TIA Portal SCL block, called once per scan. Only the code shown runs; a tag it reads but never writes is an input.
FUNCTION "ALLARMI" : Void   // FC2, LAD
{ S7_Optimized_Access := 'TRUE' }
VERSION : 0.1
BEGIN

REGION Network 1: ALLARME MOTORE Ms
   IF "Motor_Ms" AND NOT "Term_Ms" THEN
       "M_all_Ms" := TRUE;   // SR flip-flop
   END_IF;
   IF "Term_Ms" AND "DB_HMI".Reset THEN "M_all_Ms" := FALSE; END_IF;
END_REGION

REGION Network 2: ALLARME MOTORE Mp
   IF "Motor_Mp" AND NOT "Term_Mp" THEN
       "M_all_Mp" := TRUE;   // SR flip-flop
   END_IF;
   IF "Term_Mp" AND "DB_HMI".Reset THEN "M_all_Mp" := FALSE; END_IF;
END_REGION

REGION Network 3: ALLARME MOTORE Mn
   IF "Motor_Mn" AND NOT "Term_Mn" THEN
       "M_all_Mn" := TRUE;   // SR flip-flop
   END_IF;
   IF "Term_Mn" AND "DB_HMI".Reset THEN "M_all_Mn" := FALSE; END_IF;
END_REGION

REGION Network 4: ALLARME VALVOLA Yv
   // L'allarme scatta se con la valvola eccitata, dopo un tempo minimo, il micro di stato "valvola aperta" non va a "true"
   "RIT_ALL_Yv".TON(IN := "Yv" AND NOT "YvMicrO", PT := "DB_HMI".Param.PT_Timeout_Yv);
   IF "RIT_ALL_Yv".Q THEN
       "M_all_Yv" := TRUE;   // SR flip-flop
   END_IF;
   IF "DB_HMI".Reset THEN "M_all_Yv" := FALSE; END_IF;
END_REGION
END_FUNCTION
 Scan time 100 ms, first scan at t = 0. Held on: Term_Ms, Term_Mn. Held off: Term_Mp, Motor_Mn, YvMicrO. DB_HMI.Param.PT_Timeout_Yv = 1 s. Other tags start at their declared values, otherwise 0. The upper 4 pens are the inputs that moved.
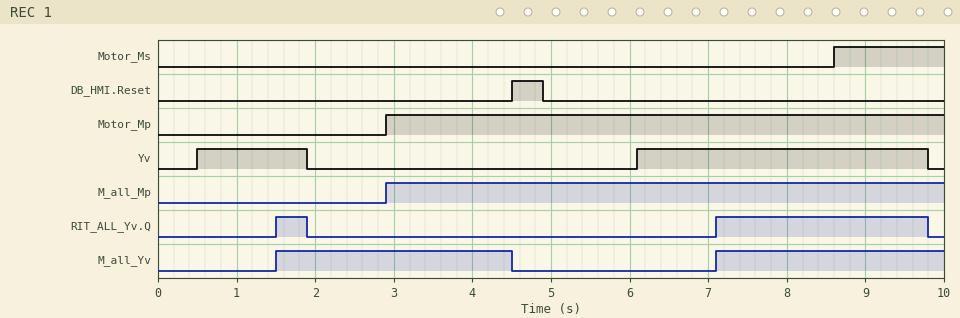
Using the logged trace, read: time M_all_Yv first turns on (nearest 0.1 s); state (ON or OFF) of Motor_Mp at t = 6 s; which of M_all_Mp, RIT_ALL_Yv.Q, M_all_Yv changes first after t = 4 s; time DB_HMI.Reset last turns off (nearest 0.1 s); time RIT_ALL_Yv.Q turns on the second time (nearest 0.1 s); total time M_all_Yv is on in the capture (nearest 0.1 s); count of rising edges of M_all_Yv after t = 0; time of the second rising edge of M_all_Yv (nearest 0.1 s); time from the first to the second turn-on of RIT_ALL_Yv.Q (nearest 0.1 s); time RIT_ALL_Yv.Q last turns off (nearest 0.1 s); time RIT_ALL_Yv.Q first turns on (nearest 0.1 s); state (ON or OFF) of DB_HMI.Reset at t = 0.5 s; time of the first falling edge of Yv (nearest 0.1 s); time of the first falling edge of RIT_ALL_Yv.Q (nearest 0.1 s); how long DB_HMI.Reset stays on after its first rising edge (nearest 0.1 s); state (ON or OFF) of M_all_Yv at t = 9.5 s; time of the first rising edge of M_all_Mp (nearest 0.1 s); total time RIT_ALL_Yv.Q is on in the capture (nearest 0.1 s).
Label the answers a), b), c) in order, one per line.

a) 1.5 s
b) ON
c) M_all_Yv
d) 4.9 s
e) 7.1 s
f) 5.9 s
g) 2
h) 7.1 s
i) 5.6 s
j) 9.8 s
k) 1.5 s
l) OFF
m) 1.9 s
n) 1.9 s
o) 0.4 s
p) ON
q) 2.9 s
r) 3.1 s
